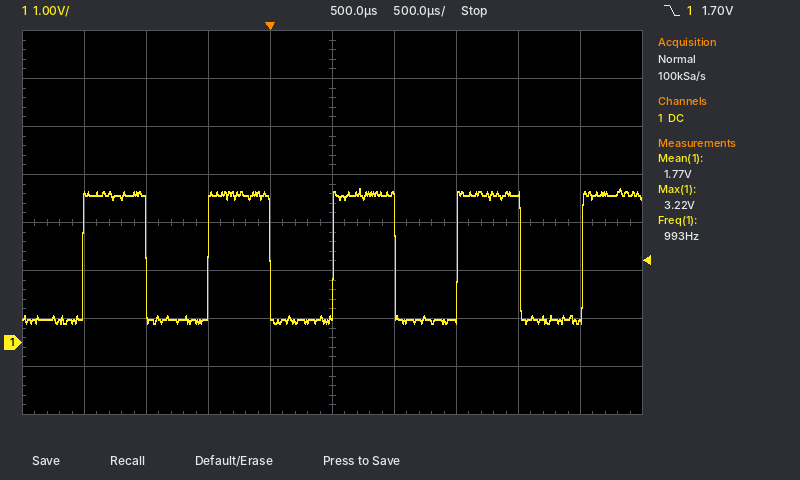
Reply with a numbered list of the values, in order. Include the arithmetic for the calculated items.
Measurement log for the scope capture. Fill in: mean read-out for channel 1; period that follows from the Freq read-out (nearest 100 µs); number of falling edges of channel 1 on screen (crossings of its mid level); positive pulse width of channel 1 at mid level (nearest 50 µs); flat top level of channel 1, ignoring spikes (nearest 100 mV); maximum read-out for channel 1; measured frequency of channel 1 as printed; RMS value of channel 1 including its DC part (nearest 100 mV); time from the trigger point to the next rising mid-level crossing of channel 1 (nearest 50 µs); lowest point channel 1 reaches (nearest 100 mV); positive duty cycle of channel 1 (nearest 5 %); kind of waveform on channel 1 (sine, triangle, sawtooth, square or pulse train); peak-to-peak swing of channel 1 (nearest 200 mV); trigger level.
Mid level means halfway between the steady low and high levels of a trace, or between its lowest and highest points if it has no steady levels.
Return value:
1. 1.77 V
2. 1 / 993 Hz ≈ 1.0 ms
3. 4
4. 500 µs
5. 3.1 V
6. 3.22 V
7. 993 Hz
8. √(0.5 × (3.1 V)² + 0.5 × (400 mV)²) ≈ 2.2 V
9. 500 µs
10. 400 mV
11. 50 %
12. square
13. 2.8 V
14. 1.70 V
